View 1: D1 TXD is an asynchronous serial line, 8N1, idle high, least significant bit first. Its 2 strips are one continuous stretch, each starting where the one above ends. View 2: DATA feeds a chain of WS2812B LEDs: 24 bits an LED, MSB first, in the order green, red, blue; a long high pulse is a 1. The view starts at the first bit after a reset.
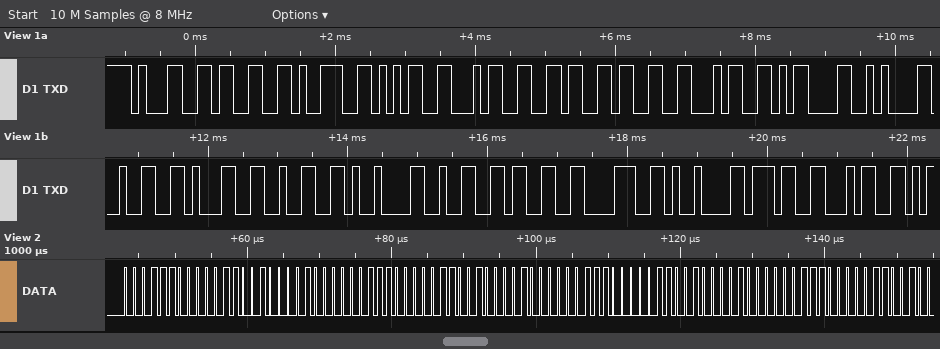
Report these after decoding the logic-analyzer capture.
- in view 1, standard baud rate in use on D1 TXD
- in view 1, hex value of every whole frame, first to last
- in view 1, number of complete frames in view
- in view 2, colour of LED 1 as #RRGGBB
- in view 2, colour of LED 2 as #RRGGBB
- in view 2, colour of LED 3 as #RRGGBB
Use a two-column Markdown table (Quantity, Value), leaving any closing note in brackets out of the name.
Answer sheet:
| Quantity | Value |
|---|---|
| in view 1, standard baud rate in use on D1 TXD | 9600 baud |
| in view 1, hex value of every whole frame, first to last | 31 33 39 35 34 36 33 34 0D 0A 32 31 32 09 32 33 38 09 37 34 |
| in view 1, number of complete frames in view | 20 |
| in view 2, colour of LED 1 as #RRGGBB | #191C08 |
| in view 2, colour of LED 2 as #RRGGBB | #191C08 |
| in view 2, colour of LED 3 as #RRGGBB | #191C08 |
